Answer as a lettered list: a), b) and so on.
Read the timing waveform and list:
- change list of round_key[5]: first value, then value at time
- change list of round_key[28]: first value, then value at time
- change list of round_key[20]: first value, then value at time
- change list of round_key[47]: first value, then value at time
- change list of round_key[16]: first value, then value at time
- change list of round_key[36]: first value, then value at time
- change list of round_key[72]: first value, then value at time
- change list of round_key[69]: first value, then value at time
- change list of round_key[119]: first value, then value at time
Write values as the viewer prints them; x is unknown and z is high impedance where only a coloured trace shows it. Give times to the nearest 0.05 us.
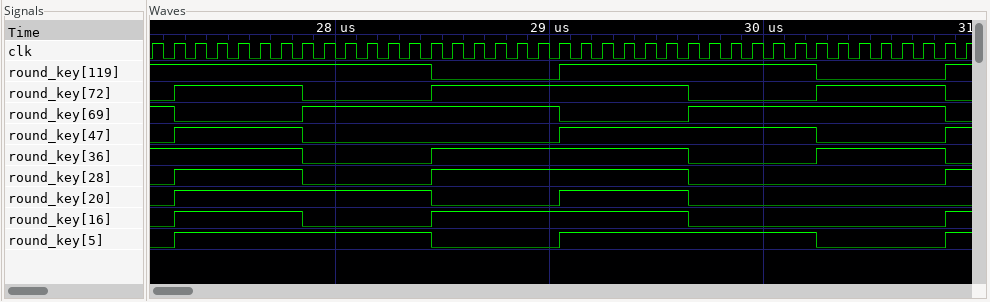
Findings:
a) 0, 1 at 27.25 us, 0 at 28.45 us, 1 at 29.05 us, 0 at 30.25 us, 1 at 30.85 us
b) 0, 1 at 27.25 us, 0 at 27.85 us, 1 at 28.45 us, 0 at 29.65 us, 1 at 30.85 us
c) 0, 1 at 27.25 us, 0 at 28.45 us, 1 at 29.05 us, 0 at 29.65 us
d) 0, 1 at 27.25 us, 0 at 27.85 us, 1 at 29.05 us, 0 at 30.25 us, 1 at 30.85 us
e) 0, 1 at 27.25 us, 0 at 27.85 us, 1 at 28.45 us, 0 at 29.65 us, 1 at 30.85 us
f) 1, 0 at 27.85 us, 1 at 28.45 us, 0 at 29.65 us, 1 at 30.25 us, 0 at 30.85 us
g) 0, 1 at 27.25 us, 0 at 27.85 us, 1 at 28.45 us, 0 at 29.65 us, 1 at 30.25 us, 0 at 30.85 us
h) 1, 0 at 27.25 us, 1 at 27.85 us, 0 at 29.05 us, 1 at 29.65 us, 0 at 30.85 us
i) 1, 0 at 28.45 us, 1 at 29.05 us, 0 at 30.25 us, 1 at 30.85 us
